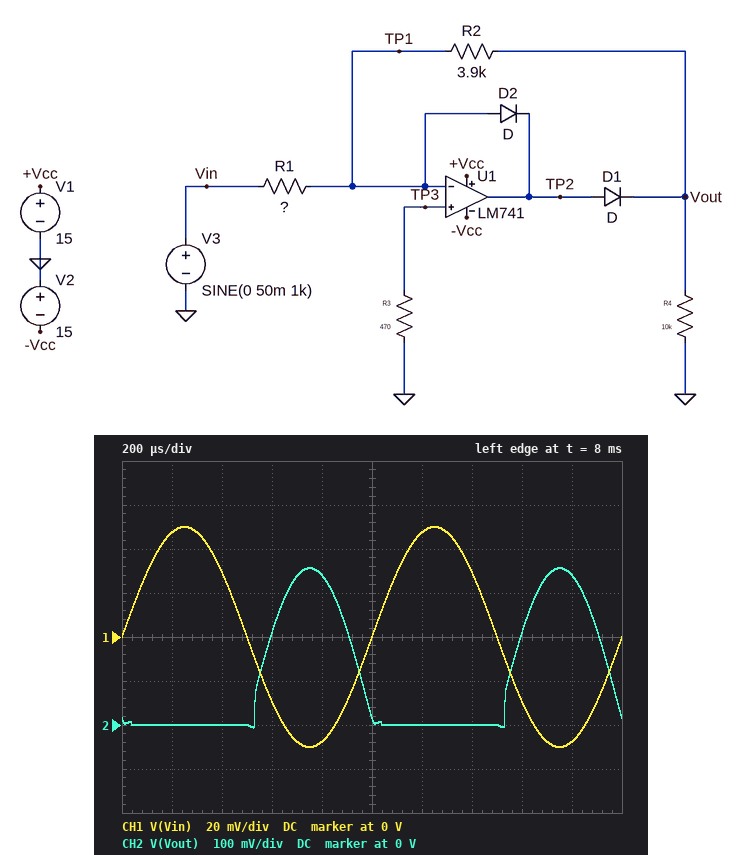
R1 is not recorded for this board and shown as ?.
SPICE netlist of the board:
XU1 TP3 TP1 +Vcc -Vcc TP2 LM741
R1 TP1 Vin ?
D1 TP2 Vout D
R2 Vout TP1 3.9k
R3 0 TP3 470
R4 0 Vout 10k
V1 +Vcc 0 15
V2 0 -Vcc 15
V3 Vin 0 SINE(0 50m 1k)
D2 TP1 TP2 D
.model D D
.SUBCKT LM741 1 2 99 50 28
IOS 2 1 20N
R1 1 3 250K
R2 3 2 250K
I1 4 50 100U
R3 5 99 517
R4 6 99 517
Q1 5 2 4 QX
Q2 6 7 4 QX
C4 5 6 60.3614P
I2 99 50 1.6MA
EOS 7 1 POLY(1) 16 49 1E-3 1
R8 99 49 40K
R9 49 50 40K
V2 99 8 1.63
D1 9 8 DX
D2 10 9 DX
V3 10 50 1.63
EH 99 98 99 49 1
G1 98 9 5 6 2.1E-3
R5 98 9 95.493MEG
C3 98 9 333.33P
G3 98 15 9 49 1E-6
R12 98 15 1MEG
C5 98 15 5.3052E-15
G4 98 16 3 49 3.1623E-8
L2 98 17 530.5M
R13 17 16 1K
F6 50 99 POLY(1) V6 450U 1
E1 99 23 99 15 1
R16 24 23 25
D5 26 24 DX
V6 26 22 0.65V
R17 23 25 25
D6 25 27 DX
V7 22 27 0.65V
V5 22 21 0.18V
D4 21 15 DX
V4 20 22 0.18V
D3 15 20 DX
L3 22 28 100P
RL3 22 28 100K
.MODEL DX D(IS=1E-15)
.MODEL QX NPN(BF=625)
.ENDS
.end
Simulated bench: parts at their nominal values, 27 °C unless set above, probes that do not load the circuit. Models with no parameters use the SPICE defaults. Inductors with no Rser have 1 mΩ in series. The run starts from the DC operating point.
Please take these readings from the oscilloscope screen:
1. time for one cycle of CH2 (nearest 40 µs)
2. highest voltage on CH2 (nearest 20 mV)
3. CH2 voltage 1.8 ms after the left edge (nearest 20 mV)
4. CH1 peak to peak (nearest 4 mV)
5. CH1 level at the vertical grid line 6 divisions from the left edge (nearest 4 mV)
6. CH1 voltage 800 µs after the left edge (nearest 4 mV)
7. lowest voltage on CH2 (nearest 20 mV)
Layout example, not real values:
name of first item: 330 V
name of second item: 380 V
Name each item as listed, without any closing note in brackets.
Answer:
time for one cycle of CH2: 1.00 ms
highest voltage on CH2: 360 mV
CH2 voltage 1.8 ms after the left edge: 340 mV
CH1 peak to peak: 100 mV
CH1 level at the vertical grid line 6 divisions from the left edge: 48 mV
CH1 voltage 800 µs after the left edge: -48 mV
lowest voltage on CH2: 0 V
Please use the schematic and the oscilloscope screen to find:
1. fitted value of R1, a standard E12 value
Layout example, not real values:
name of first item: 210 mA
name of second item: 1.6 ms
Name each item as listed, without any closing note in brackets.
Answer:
fitted value of R1, a standard E12 value: 560 Ω
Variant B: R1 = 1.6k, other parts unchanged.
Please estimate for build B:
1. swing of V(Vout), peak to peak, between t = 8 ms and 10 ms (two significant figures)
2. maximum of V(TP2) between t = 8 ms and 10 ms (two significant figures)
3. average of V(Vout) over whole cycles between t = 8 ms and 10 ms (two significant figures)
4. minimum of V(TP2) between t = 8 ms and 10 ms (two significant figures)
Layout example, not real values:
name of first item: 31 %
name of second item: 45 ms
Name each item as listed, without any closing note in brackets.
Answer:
swing of V(Vout), peak to peak, between t = 8 ms and 10 ms: 130 mV
maximum of V(TP2) between t = 8 ms and 10 ms: 700 mV
average of V(Vout) over whole cycles between t = 8 ms and 10 ms: 41 mV
minimum of V(TP2) between t = 8 ms and 10 ms: -560 mV
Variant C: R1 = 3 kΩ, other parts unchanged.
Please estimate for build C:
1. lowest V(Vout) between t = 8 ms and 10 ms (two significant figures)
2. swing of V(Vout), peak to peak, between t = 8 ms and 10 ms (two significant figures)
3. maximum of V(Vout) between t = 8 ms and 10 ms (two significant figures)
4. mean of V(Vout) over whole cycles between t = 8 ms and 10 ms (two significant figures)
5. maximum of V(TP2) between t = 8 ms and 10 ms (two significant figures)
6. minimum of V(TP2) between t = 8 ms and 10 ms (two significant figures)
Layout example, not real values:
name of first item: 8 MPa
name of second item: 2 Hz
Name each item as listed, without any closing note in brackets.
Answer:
lowest V(Vout) between t = 8 ms and 10 ms: -5.0 mV
swing of V(Vout), peak to peak, between t = 8 ms and 10 ms: 73 mV
maximum of V(Vout) between t = 8 ms and 10 ms: 68 mV
mean of V(Vout) over whole cycles between t = 8 ms and 10 ms: 22 mV
maximum of V(TP2) between t = 8 ms and 10 ms: 630 mV
minimum of V(TP2) between t = 8 ms and 10 ms: -550 mV
